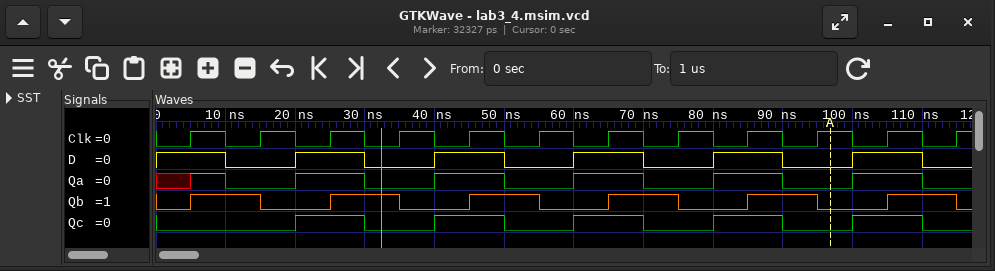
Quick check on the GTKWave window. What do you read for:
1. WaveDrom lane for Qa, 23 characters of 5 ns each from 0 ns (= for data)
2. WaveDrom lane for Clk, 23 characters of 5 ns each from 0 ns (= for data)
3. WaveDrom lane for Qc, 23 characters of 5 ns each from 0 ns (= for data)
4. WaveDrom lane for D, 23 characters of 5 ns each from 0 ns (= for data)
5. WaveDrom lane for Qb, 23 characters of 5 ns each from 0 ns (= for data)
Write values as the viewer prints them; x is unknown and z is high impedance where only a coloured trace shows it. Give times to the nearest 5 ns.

{name: 'Qa', wave: 'x10.1.0.1.0.1.0.1.0.1.0'}
{name: 'Clk', wave: '01010101010101010101010'}
{name: 'Qc', wave: '0...1.0.1.0.1.0.1.0.1.0'}
{name: 'D', wave: '1.0.1.0.1.0.1.0.1.0.1.0'}
{name: 'Qb', wave: '01.0.1.0.1.0.1.0.1.0.1.'}
